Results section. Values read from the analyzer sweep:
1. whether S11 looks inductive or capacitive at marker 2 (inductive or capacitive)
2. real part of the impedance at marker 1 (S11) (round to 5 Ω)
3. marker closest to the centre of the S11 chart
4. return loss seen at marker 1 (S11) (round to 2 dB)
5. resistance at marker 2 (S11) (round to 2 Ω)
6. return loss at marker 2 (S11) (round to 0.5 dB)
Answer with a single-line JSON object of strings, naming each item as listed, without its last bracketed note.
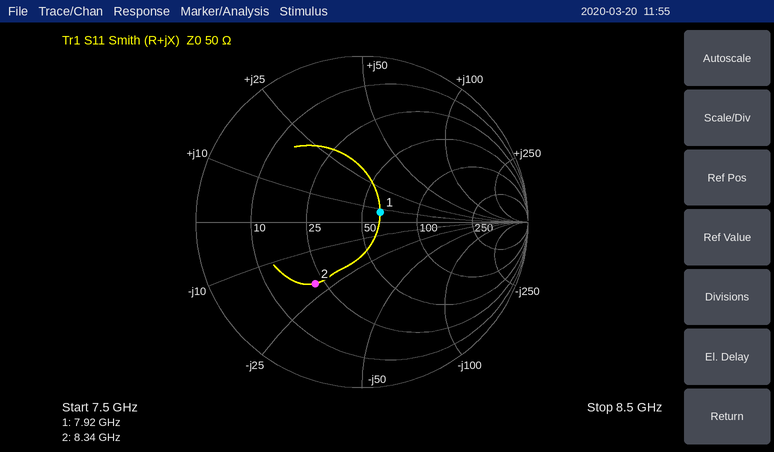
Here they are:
{"whether S11 looks inductive or capacitive at marker 2": "capacitive", "real part of the impedance at marker 1 (S11)": "60 Ω", "marker closest to the centre of the S11 chart": "marker 1", "return loss seen at marker 1 (S11)": "18 dB", "resistance at marker 2 (S11)": "22 Ω", "return loss at marker 2 (S11)": "6.5 dB"}
